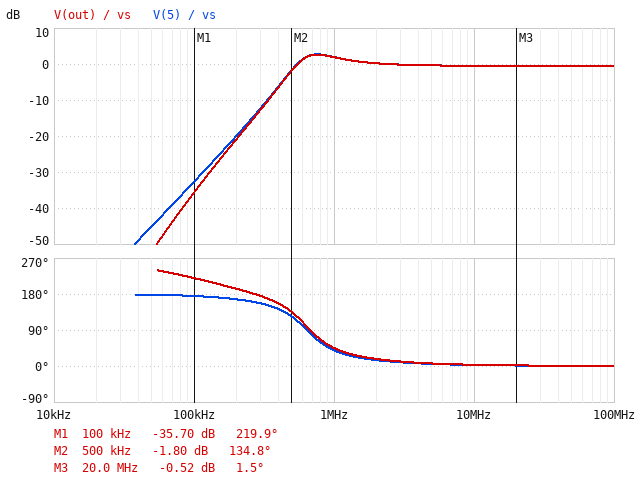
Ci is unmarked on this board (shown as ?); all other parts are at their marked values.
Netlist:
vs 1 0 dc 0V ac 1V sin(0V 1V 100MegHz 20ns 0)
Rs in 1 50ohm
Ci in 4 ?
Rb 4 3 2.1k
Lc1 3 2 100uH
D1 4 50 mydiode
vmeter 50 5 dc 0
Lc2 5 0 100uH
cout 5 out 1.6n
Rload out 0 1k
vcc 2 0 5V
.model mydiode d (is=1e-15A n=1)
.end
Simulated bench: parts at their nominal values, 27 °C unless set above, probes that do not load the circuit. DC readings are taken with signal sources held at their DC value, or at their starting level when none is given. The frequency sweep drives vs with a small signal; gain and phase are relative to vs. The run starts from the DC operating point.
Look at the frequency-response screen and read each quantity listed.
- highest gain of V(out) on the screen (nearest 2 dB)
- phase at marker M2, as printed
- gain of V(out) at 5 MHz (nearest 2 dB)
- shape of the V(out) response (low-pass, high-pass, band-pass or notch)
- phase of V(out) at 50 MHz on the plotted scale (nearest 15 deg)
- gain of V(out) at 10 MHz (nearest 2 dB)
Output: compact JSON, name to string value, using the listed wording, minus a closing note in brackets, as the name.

{"highest gain of V(out) on the screen": "2 dB", "phase at marker M2, as printed": "134.8 deg", "gain of V(out) at 5 MHz": "0 dB", "shape of the V(out) response": "high-pass", "phase of V(out) at 50 MHz on the plotted scale": "0 deg", "gain of V(out) at 10 MHz": "0 dB"}
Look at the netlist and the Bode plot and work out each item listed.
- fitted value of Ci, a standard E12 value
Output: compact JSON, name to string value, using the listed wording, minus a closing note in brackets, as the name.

{"fitted value of Ci, a standard E12 value": "560 pF"}
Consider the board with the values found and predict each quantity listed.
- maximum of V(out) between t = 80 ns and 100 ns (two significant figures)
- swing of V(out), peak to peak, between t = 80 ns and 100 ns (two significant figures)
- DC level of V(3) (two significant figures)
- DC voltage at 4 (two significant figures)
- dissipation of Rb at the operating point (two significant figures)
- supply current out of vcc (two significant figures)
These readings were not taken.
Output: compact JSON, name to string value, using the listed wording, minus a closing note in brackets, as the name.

{"maximum of V(out) between t = 80 ns and 100 ns": "940 mV", "swing of V(out), peak to peak, between t = 80 ns and 100 ns": "1.9 V", "DC level of V(3)": "5.0 V", "DC voltage at 4": "730 mV", "dissipation of Rb at the operating point": "8.7 mW", "supply current out of vcc": "2.0 mA"}
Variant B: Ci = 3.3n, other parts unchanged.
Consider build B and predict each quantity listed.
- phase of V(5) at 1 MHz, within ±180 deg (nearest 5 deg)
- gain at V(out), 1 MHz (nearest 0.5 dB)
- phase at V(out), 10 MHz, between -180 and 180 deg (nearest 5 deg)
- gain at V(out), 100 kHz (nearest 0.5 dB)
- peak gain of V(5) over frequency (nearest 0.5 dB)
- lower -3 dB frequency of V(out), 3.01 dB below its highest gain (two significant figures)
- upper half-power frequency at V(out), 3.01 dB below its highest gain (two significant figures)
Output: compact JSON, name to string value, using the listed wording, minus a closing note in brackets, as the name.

{"phase of V(5) at 1 MHz, within ±180 deg": "10 deg", "gain at V(out), 1 MHz": "0 dB", "phase at V(out), 10 MHz, between -180 and 180 deg": "0 deg", "gain at V(out), 100 kHz": "-19.5 dB", "peak gain of V(5) over frequency": "4.5 dB", "lower -3 dB frequency of V(out), 3.01 dB below its highest gain": "220 kHz", "upper half-power frequency at V(out), 3.01 dB below its highest gain": "520 kHz"}
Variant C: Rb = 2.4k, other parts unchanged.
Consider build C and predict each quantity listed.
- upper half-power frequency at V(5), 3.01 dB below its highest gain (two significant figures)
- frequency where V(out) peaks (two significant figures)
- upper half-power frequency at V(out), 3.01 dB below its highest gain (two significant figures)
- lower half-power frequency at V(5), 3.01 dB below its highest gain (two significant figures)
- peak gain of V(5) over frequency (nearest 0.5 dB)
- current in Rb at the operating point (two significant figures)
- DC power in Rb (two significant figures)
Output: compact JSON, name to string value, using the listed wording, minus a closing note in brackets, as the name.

{"upper half-power frequency at V(5), 3.01 dB below its highest gain": "2.9 MHz", "frequency where V(out) peaks": "750 kHz", "upper half-power frequency at V(out), 3.01 dB below its highest gain": "3.2 MHz", "lower half-power frequency at V(5), 3.01 dB below its highest gain": "530 kHz", "peak gain of V(5) over frequency": "3.0 dB", "current in Rb at the operating point": "1.8 mA", "DC power in Rb": "7.6 mW"}
